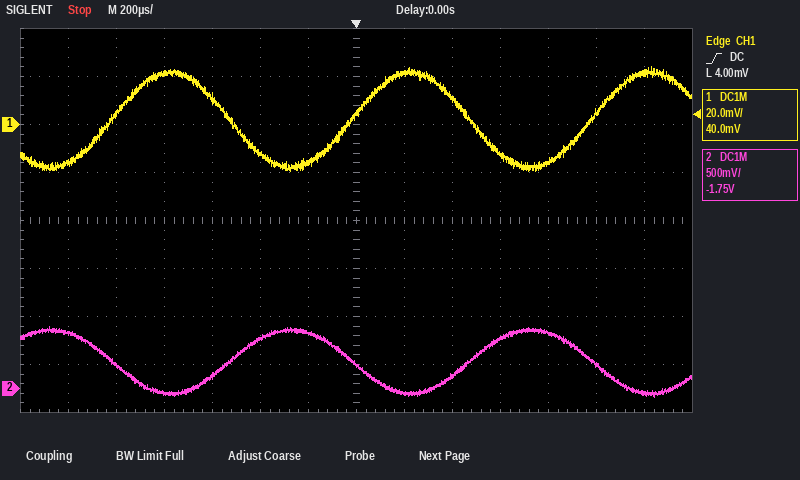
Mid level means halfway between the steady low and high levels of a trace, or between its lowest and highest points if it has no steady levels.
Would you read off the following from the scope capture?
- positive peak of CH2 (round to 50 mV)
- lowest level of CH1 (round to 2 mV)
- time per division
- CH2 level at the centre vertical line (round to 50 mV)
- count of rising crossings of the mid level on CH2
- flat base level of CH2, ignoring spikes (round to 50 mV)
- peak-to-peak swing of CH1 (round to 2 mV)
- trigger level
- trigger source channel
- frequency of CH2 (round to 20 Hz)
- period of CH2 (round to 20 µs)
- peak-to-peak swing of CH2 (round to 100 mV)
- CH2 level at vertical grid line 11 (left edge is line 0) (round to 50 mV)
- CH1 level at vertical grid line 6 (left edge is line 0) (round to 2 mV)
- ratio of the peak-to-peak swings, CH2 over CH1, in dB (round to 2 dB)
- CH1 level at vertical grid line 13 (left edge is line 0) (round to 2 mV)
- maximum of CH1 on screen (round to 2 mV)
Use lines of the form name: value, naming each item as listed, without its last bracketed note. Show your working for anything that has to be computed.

positive peak of CH2: 650 mV
lowest level of CH1: -20 mV
time per division: 200 µs
CH2 level at the centre vertical line: 250 mV
count of rising crossings of the mid level on CH2: 2
flat base level of CH2, ignoring spikes: -50 mV
peak-to-peak swing of CH1: 24 mV − (-20 mV) = 44 mV
trigger level: 4.00 mV
trigger source channel: CH1
frequency of CH2: 1 / 1.00 ms ≈ 1.00 kHz
period of CH2: 1.00 ms
peak-to-peak swing of CH2: 700 mV
CH2 level at vertical grid line 11 (left edge is line 0): 600 mV
CH1 level at vertical grid line 6 (left edge is line 0): -16 mV
ratio of the peak-to-peak swings, CH2 over CH1, in dB: 20 log10(700 mV / 44 mV) ≈ 24 dB
CH1 level at vertical grid line 13 (left edge is line 0): 22 mV
maximum of CH1 on screen: 24 mV
